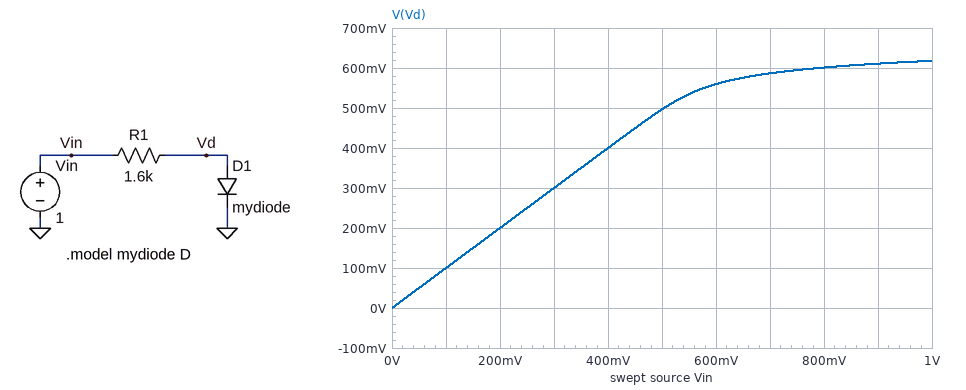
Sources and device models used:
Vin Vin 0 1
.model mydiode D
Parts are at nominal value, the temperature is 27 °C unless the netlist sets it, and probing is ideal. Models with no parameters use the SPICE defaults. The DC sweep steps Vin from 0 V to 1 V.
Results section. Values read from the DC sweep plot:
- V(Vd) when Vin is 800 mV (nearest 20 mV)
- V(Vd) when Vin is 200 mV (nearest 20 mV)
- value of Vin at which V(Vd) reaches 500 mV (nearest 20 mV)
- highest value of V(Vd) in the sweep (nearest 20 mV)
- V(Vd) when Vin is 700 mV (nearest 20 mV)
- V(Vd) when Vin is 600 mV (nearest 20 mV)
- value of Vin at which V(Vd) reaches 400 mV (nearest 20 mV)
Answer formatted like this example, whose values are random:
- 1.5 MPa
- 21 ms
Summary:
- 600 mV
- 200 mV
- 500 mV
- 620 mV
- 580 mV
- 560 mV
- 400 mV
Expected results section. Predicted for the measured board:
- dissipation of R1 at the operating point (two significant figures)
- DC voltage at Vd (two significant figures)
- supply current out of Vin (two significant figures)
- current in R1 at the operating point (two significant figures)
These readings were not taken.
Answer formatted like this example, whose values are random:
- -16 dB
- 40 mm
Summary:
- 91 µW
- 620 mV
- 240 µA
- 240 µA
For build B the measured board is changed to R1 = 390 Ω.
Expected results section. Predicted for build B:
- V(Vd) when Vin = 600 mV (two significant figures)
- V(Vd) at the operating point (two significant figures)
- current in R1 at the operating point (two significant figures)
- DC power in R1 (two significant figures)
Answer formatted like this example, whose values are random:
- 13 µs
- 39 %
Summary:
- 580 mV
- 650 mV
- 890 µA
- 310 µW
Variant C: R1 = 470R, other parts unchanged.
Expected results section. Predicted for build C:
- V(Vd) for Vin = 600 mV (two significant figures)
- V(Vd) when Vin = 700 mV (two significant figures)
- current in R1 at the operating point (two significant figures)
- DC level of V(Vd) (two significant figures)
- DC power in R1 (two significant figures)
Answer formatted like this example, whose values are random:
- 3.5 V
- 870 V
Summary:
- 580 mV
- 610 mV
- 750 µA
- 650 mV
- 260 µW
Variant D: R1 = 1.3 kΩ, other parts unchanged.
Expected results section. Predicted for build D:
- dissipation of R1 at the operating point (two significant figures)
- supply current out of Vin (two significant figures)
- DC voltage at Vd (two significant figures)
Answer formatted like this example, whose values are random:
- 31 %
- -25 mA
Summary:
- 110 µW
- 290 µA
- 620 mV
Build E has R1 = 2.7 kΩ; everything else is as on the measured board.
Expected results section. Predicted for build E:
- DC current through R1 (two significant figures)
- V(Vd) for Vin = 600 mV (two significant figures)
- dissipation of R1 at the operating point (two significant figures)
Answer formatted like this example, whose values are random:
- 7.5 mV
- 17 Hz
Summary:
- 150 µA
- 550 mV
- 58 µW
